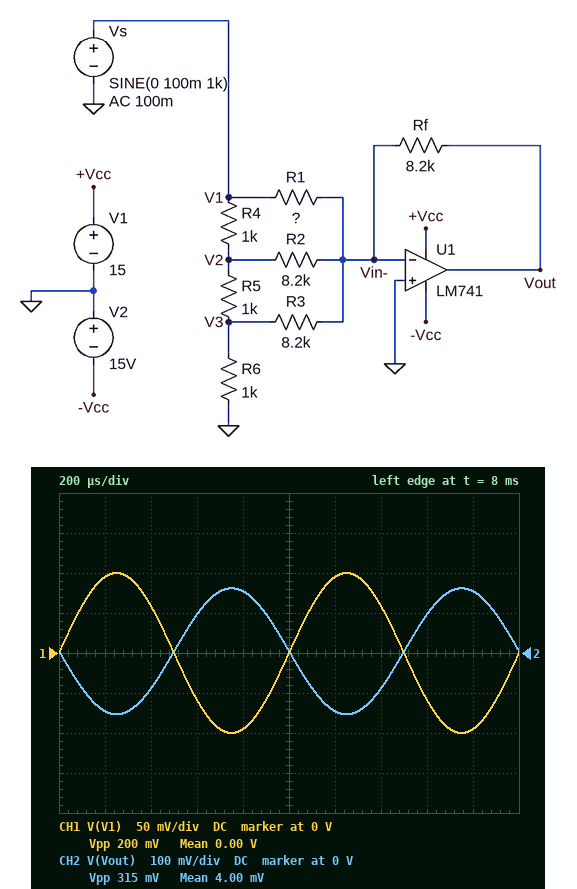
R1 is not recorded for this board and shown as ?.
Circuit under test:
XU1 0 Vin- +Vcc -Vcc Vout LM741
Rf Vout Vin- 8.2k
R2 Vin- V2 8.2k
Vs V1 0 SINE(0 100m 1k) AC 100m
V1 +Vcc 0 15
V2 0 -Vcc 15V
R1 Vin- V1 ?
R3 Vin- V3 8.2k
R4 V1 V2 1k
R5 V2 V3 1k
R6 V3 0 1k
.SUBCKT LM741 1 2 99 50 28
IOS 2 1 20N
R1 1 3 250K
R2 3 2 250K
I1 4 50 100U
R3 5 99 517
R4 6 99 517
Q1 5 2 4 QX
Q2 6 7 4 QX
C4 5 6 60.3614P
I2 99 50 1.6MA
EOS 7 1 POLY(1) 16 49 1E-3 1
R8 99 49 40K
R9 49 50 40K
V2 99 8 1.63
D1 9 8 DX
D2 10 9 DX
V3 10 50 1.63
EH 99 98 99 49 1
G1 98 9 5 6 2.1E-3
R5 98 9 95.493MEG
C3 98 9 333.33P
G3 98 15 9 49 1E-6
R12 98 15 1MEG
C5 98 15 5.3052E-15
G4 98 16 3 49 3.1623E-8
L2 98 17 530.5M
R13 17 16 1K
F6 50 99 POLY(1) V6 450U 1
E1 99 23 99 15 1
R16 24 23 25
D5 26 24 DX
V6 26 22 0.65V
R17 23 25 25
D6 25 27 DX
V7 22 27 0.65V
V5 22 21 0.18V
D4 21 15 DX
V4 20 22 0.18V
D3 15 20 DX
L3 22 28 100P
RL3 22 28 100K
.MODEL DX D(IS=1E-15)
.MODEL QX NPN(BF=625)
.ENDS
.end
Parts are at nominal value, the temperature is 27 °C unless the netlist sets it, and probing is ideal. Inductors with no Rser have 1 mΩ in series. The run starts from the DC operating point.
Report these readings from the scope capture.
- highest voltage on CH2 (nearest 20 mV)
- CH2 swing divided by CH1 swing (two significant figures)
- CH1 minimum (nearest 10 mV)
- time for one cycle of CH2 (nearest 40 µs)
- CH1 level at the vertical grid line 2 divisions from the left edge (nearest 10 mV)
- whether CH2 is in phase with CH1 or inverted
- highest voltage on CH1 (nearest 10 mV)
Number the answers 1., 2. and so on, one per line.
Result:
1. 160 mV
2. 1.6
3. -100 mV
4. 1.00 ms
5. 60 mV
6. inverted
7. 100 mV
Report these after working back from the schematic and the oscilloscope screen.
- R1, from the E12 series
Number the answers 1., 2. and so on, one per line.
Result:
1. 12 kΩ
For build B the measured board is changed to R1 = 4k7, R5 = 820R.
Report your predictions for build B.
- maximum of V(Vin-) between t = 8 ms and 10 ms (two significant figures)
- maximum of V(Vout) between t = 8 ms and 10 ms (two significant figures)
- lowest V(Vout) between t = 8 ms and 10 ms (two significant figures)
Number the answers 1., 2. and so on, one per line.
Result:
1. 1.3 mV
2. 270 mV
3. -260 mV
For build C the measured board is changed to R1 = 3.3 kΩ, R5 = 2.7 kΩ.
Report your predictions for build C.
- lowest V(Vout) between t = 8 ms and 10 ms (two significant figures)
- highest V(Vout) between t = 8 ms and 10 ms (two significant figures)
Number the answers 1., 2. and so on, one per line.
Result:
1. -330 mV
2. 340 mV
